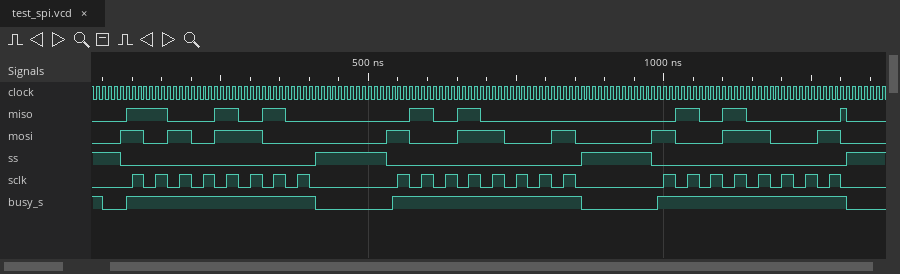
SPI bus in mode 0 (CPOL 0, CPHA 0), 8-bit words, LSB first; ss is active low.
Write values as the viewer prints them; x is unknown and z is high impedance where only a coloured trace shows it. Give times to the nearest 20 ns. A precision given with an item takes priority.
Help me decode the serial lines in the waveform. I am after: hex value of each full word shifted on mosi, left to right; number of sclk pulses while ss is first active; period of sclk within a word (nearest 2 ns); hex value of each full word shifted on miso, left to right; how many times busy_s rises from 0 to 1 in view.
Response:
35, 99, 99
8
40 ns
53, 0A, 0A
3
